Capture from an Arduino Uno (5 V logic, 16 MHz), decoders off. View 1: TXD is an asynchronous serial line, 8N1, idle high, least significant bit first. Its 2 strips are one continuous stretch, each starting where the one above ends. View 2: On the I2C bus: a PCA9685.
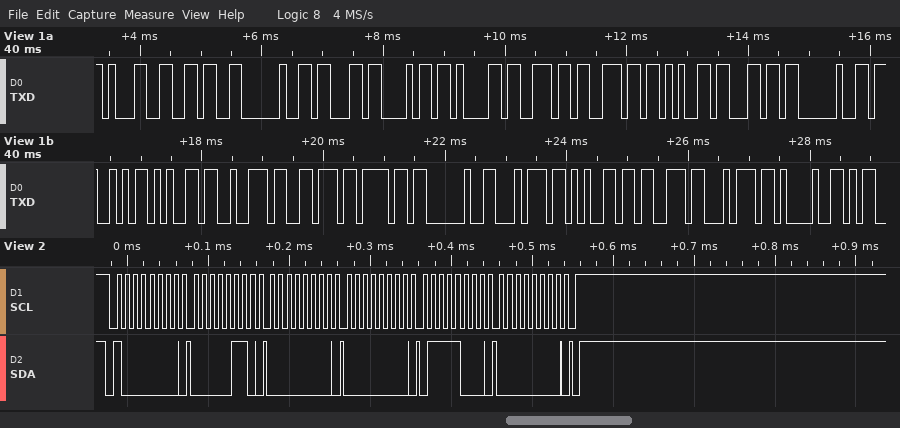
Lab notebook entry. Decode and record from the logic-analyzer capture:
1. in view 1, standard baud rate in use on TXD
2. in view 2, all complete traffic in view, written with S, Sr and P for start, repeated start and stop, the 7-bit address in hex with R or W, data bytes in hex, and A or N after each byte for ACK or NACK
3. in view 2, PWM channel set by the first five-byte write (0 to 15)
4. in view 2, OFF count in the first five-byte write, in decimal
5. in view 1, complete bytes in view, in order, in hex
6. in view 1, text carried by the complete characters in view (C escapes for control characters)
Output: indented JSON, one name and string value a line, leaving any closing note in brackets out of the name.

{
  "in view 1, standard baud rate in use on TXD": "9600 baud",
  "in view 2, all complete traffic in view, written with S, Sr and P for start, repeated start and stop, the 7-bit address in hex with R or W, data bytes in hex, and A or N after each byte for ACK or NACK": "S 40W A 06 A 00 A 00 A 78 A 00 A P",
  "in view 2, PWM channel set by the first five-byte write": "0",
  "in view 2, OFF count in the first five-byte write, in decimal": "120",
  "in view 1, complete bytes in view, in order, in hex": "31 36 20 63 68 61 6E 6E 65 6C 20 53 65 72 76 6F 20 74 65 73 74 21",
  "in view 1, text carried by the complete characters in view": "\"16 channel Servo test!\""
}
